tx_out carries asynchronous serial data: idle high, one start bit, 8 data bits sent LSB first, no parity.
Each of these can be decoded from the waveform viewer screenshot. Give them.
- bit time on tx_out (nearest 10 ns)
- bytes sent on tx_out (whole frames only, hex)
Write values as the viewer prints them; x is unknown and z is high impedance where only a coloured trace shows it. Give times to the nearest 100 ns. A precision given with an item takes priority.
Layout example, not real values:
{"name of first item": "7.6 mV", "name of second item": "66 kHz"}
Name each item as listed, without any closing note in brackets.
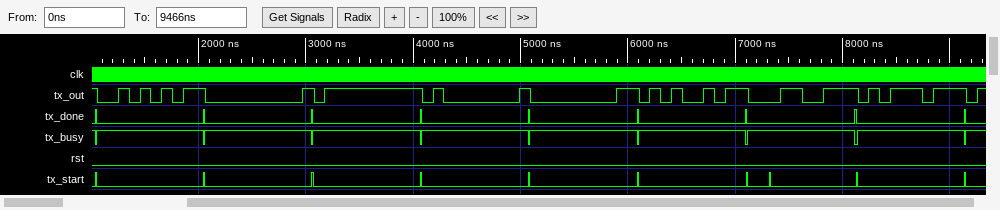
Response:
{"bit time on tx_out": "100 ns", "bytes sent on tx_out": "AA, 00, FF, 01, 80, A5, CC, DD"}
